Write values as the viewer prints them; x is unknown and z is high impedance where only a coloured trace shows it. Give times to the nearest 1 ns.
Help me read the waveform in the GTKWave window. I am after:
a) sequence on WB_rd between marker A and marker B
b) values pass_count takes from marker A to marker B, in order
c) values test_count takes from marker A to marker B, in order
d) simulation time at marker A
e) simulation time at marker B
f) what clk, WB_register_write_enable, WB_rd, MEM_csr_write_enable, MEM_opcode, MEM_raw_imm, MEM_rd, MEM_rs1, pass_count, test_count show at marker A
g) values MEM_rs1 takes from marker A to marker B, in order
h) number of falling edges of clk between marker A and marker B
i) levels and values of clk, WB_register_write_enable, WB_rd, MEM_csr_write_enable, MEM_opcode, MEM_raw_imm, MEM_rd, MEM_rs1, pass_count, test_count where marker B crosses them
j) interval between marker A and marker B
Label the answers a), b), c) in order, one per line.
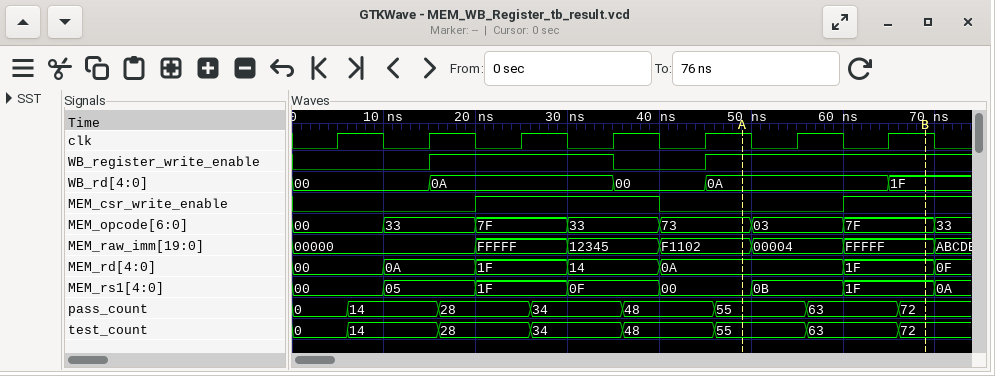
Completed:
a) 0A, 1F
b) 55, 63, 72
c) 55, 63, 72
d) 49 ns
e) 69 ns
f) clk=1, WB_register_write_enable=1, WB_rd=0A, MEM_csr_write_enable=0, MEM_opcode=73, MEM_raw_imm=F1102, MEM_rd=0A, MEM_rs1=00, pass_count=55, test_count=55
g) 00, 0B, 1F
h) 2
i) clk=1, WB_register_write_enable=1, WB_rd=1F, MEM_csr_write_enable=1, MEM_opcode=7F, MEM_raw_imm=FFFFF, MEM_rd=1F, MEM_rs1=1F, pass_count=72, test_count=72
j) 20 ns
